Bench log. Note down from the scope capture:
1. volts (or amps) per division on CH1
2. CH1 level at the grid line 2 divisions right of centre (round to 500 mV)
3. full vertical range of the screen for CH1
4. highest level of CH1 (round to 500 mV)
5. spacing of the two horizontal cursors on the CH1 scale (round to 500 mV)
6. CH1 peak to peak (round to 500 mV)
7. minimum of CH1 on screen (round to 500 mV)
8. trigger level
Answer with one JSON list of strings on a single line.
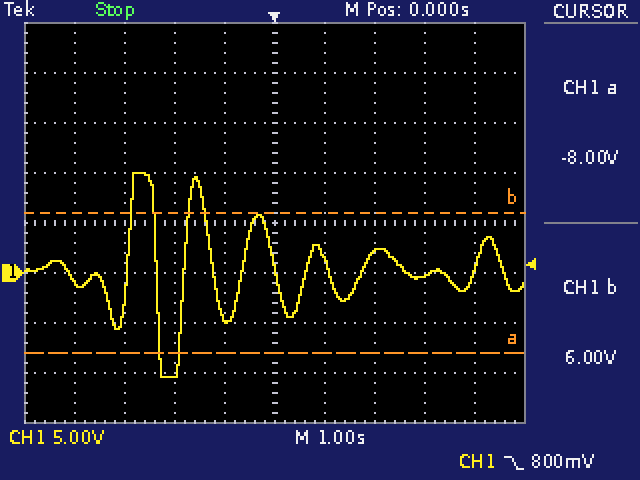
["5 V", "2.0 V", "40 V", "10.0 V", "14.0 V", "20.5 V", "-10.5 V", "800 mV"]
